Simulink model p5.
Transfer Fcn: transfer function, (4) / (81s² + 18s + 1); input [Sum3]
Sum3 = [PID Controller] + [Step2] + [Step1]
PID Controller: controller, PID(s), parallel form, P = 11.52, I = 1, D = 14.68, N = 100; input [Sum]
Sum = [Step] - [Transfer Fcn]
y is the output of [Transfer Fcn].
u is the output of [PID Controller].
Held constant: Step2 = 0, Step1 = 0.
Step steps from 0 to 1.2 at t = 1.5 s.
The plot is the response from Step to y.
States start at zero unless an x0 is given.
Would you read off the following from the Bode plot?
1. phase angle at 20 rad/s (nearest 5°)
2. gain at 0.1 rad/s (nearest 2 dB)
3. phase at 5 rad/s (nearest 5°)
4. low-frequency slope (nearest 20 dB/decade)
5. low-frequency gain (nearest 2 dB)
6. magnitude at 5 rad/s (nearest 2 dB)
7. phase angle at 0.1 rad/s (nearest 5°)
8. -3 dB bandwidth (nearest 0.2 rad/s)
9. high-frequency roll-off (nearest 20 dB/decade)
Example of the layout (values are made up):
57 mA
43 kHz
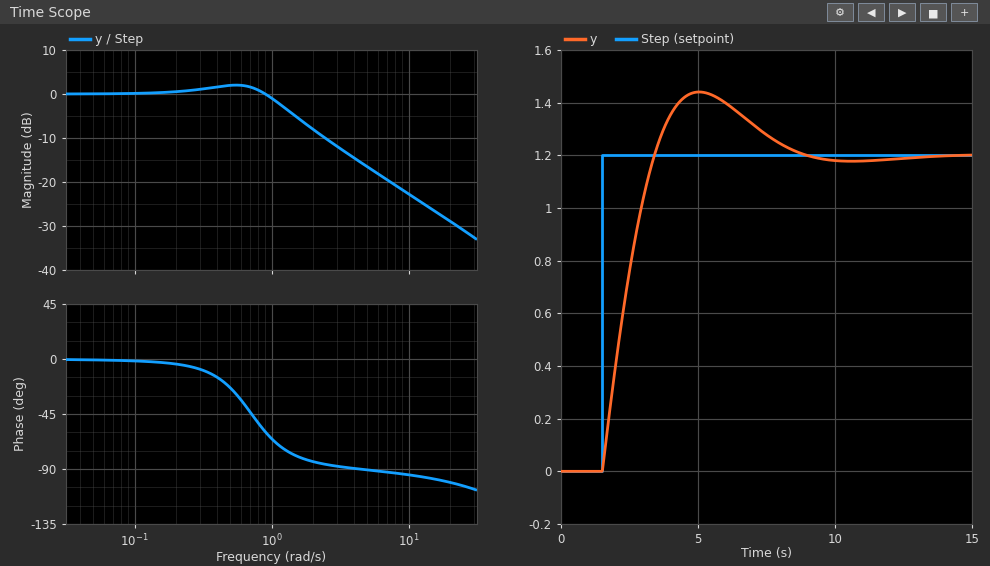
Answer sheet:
-100°
0 dB
-90°
0 dB/decade
0 dB
-16 dB
0°
1.2 rad/s
-20 dB/decade
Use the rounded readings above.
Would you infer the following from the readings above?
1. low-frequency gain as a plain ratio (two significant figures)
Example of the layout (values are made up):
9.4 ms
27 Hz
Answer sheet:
1.0
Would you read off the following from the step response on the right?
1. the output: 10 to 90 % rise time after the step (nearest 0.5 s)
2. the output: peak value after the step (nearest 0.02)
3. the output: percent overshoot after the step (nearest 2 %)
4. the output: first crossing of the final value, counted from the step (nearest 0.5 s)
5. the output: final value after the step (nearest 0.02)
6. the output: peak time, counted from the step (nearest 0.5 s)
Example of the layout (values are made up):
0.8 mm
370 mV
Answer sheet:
1.5 s
1.44
20 %
2.0 s
1.20
3.5 s
